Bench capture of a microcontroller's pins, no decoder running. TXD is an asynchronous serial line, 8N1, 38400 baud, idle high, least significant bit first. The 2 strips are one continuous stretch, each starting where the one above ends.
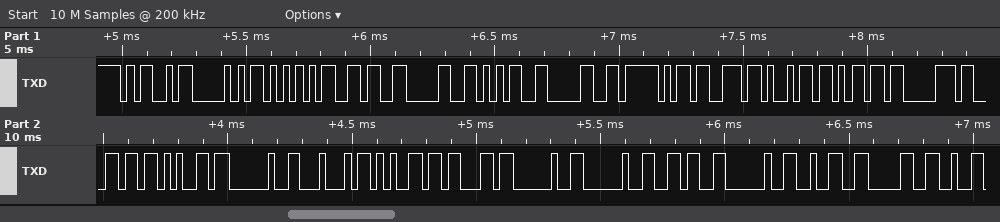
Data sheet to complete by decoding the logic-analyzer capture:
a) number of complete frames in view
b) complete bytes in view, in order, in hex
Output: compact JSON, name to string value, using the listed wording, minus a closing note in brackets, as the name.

{"number of complete frames in view": "24", "complete bytes in view, in order, in hex": "4D 50 55 36 30 35 30 5F 73 69 6D 70 6C 65 20 44 65 63 20 20 36 20 32 30"}
